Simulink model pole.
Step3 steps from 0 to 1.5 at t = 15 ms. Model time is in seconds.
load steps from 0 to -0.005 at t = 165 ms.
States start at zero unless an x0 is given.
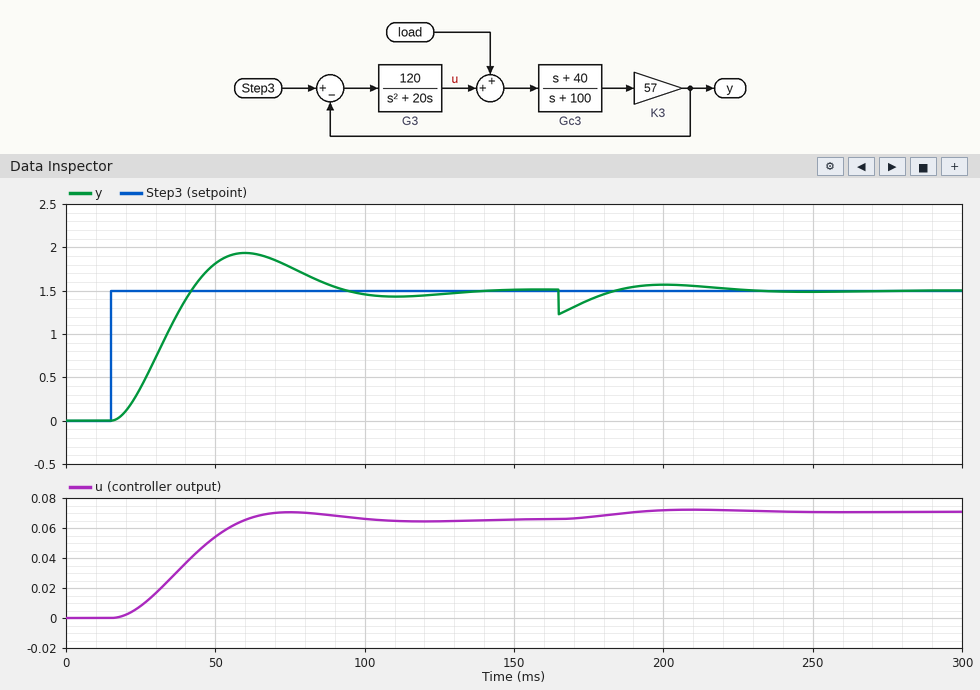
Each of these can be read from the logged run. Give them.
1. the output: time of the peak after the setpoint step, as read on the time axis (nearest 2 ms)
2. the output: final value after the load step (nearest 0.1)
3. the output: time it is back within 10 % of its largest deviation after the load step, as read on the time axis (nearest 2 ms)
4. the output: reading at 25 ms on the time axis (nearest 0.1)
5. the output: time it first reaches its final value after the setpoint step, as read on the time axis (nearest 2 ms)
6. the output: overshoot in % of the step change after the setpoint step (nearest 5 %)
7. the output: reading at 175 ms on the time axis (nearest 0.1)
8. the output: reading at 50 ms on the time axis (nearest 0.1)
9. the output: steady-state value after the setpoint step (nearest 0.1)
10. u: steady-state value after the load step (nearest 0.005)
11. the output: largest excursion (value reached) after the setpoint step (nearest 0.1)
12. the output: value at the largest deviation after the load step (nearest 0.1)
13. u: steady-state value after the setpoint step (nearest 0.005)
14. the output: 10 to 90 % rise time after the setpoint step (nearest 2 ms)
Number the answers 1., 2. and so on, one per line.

1. 60 ms
2. 1.5
3. 220 ms
4. 0.4
5. 42 ms
6. 30 %
7. 1.4
8. 1.8
9. 1.5
10. 0.070
11. 1.9
12. 1.2
13. 0.065
14. 18 ms
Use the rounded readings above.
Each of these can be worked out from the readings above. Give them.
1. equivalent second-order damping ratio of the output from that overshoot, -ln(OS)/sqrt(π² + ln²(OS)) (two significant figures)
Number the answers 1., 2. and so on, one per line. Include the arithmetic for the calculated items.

1. ln(0.3) = -1.204; 1.204 / sqrt(9.870 + 1.450) = 0.36
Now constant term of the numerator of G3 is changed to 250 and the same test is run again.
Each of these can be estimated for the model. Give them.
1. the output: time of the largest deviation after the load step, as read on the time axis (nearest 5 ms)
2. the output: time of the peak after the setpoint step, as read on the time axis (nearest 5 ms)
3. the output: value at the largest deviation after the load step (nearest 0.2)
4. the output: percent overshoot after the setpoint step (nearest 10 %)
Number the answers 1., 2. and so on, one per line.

1. 165 ms
2. 45 ms
3. 1.2
4. 40 %
